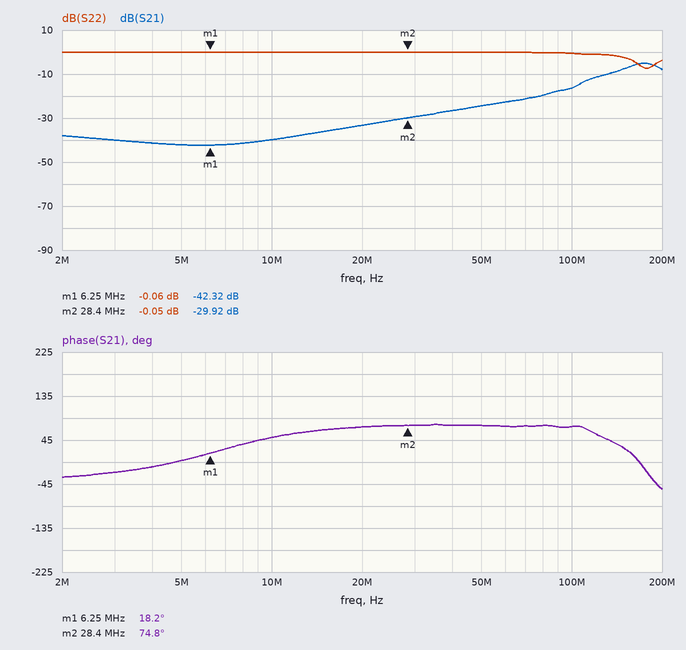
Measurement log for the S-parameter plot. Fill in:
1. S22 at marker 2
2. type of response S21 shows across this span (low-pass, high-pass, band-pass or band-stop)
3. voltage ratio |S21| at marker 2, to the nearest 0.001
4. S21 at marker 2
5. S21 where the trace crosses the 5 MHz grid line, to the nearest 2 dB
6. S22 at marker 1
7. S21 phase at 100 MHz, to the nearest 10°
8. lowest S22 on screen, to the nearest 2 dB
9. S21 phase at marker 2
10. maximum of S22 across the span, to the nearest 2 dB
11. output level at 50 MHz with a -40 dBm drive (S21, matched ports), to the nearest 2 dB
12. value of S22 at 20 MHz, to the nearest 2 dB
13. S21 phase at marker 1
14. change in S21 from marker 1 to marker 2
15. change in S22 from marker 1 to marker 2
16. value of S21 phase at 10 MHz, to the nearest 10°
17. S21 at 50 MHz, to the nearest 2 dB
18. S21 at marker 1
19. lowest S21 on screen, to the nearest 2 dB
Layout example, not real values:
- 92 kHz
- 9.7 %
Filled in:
- -0.05 dB
- high-pass
- 0.032
- -29.92 dB
- -42 dB
- -0.06 dB
- 70°
- -8 dB
- 74.8°
- 0 dB
- -64 dBm
- 0 dB
- 18.2°
- 12.40 dB
- 0.01 dB
- 50°
- -24 dB
- -42.32 dB
- -42 dB
